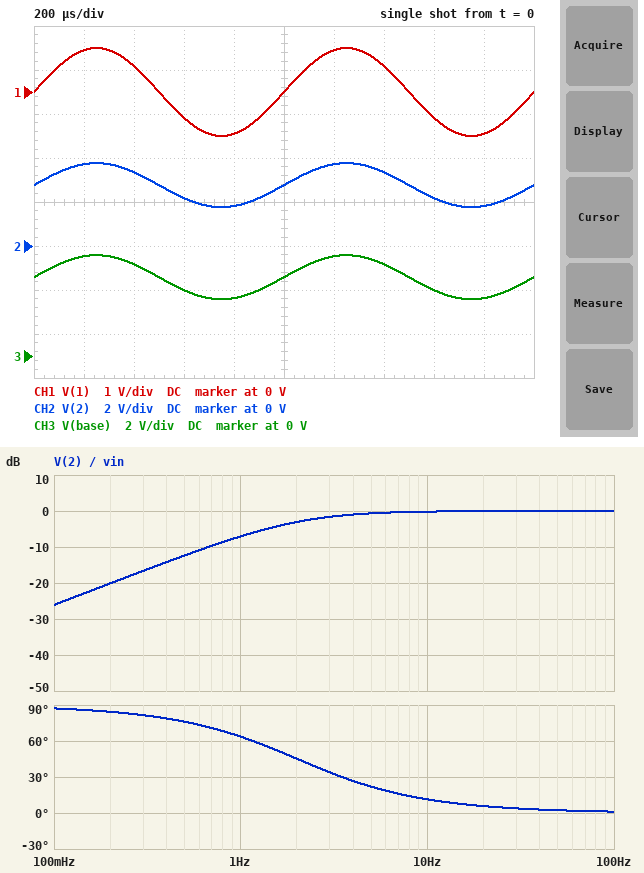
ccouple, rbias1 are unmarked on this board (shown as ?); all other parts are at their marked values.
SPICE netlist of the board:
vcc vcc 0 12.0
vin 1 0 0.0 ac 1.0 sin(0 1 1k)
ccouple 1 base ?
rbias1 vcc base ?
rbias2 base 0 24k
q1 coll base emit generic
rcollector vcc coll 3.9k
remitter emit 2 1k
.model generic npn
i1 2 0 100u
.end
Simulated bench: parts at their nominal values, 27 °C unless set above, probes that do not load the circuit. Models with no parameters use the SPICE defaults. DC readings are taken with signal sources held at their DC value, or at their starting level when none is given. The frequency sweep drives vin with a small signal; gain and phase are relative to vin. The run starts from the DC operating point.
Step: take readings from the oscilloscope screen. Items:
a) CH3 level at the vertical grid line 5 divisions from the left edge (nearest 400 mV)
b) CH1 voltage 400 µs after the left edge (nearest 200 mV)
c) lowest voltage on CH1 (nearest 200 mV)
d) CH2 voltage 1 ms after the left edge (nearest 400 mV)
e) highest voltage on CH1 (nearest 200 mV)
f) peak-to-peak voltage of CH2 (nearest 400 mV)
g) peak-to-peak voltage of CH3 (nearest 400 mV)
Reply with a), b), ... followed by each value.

a) 3.6 V
b) 600 mV
c) -1.0 V
d) 2.8 V
e) 1.0 V
f) 2.0 V
g) 2.0 V
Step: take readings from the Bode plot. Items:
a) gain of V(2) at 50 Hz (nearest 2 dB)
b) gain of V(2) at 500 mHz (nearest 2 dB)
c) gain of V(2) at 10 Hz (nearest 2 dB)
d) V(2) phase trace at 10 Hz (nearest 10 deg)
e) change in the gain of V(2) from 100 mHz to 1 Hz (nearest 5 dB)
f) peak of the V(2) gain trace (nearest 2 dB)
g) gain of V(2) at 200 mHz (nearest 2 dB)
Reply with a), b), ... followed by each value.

a) 0 dB
b) -12 dB
c) 0 dB
d) 10 deg
e) 20 dB
f) 0 dB
g) -20 dB
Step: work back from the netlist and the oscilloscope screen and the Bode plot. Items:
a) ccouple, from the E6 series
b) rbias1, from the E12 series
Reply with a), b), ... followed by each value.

a) 4.7 µF
b) 56 kΩ
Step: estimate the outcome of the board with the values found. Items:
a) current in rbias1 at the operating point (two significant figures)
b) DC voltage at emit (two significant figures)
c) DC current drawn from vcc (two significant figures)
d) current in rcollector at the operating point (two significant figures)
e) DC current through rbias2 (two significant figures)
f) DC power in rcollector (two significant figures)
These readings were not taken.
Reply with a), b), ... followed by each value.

a) 150 µA
b) 2.9 V
c) 250 µA
d) 99 µA
e) 150 µA
f) 38 µW
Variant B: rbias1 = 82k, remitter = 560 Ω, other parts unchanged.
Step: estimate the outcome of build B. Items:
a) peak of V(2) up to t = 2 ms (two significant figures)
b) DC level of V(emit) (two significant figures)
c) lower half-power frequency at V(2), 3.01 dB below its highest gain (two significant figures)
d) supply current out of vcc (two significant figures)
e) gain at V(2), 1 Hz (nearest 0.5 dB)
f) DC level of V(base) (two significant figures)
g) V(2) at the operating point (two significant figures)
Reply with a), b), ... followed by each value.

a) 2.9 V
b) 2.0 V
c) 1.8 Hz
d) 210 µA
e) -6.5 dB
f) 2.7 V
g) 1.9 V
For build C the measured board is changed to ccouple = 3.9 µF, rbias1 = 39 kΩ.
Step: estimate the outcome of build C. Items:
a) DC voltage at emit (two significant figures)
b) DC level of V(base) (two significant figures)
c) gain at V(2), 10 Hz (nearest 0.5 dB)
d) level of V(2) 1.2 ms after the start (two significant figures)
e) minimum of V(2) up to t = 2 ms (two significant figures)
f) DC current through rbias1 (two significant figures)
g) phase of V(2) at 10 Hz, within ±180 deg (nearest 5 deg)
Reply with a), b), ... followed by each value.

a) 3.8 V
b) 4.6 V
c) -0.5 dB
d) 4.7 V
e) 2.7 V
f) 190 µA
g) 15 deg
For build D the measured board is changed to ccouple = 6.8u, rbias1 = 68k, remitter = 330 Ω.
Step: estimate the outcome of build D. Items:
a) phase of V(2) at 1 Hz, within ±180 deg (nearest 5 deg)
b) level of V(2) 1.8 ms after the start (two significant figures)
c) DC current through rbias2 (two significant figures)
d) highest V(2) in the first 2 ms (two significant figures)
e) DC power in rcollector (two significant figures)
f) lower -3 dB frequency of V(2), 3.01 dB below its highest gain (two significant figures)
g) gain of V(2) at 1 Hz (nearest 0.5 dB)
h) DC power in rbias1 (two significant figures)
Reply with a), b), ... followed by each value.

a) 55 deg
b) 1.4 V
c) 130 µA
d) 3.4 V
e) 38 µW
f) 1.3 Hz
g) -4.5 dB
h) 1.2 mW
